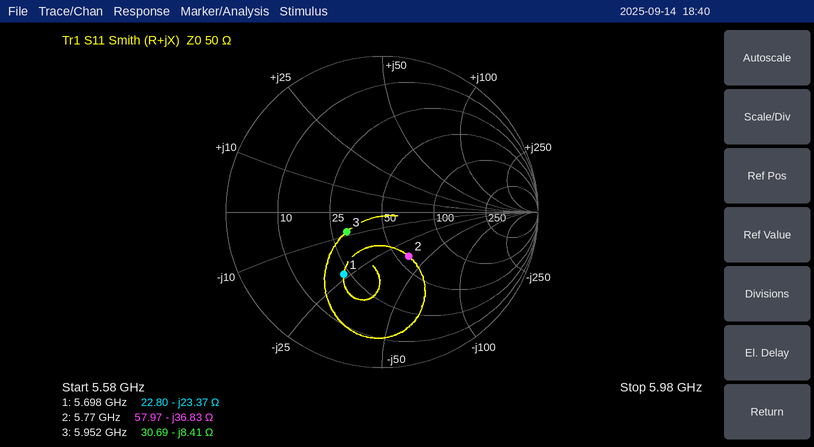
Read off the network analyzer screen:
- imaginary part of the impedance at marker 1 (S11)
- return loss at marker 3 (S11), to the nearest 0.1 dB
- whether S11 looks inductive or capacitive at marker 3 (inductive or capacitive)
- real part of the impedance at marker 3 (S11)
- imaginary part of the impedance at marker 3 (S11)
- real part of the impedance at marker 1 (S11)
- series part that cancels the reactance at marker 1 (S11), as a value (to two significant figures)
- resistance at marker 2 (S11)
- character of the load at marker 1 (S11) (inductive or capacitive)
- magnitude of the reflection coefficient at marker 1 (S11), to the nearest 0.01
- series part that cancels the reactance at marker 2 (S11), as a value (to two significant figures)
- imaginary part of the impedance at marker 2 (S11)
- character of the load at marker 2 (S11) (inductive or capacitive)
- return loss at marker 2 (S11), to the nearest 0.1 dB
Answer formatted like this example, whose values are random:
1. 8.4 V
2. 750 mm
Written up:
1. -23.37 Ω
2. 11.7 dB
3. capacitive
4. 30.69 Ω
5. -8.41 Ω
6. 22.80 Ω
7. 650 pH
8. 57.97 Ω
9. capacitive
10. 0.47
11. 1.0 nH
12. -36.83 Ω
13. capacitive
14. 9.6 dB
